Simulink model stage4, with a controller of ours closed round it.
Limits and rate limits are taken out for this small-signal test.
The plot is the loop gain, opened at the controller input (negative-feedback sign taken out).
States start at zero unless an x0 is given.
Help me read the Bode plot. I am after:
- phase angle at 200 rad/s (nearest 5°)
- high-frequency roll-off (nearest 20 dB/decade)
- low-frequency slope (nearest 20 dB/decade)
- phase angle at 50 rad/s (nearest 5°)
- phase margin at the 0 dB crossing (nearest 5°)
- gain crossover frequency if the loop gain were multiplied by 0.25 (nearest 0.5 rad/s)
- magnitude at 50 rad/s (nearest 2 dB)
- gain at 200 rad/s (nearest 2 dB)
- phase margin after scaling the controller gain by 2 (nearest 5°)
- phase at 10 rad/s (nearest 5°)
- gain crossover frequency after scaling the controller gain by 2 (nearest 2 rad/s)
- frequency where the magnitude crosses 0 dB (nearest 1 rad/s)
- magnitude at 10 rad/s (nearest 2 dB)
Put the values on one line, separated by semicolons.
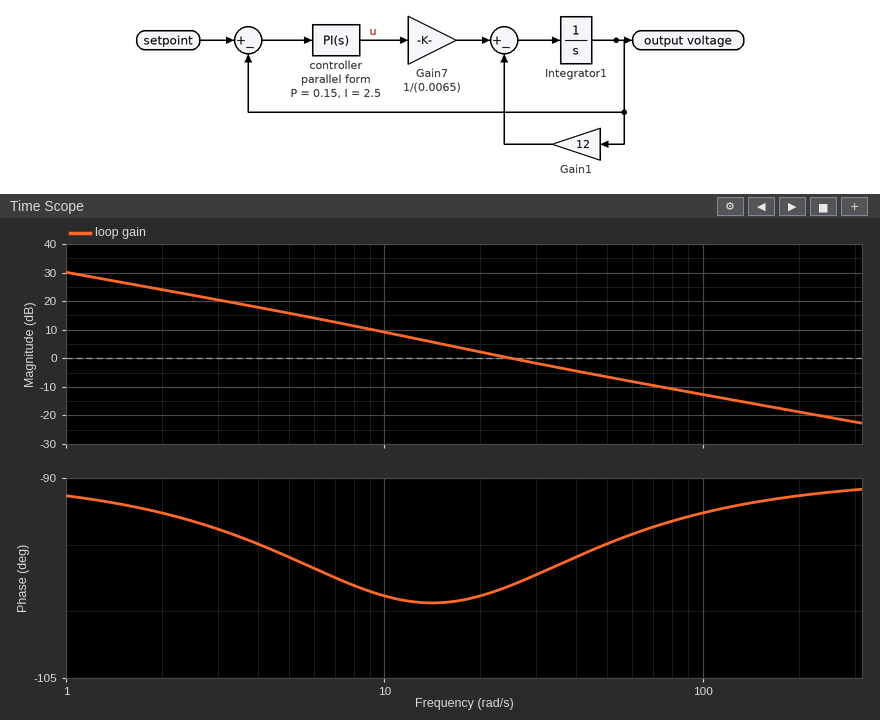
-90°; -20 dB/decade; -20 dB/decade; -95°; 80°; 7.5 rad/s; -6 dB; -18 dB; 85°; -100°; 48 rad/s; 25 rad/s; 10 dB
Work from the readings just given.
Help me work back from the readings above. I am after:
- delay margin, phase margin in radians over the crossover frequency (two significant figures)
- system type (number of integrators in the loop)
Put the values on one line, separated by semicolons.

0.056 s; 1
